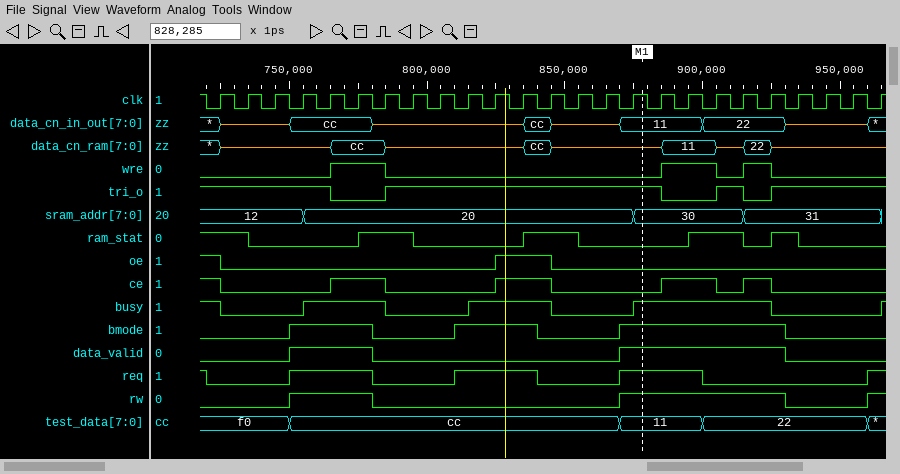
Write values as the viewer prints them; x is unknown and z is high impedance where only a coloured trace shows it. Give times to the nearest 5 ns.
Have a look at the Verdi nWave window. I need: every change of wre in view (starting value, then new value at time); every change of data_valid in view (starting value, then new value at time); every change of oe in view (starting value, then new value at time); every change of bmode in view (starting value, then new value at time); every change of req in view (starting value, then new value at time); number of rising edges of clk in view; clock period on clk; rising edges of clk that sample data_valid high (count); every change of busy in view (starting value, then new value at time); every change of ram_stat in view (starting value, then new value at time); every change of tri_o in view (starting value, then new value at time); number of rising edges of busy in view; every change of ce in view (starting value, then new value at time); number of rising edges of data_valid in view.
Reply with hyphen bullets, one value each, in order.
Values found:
- 0, 1 at 765 ns, 0 at 785 ns, 1 at 885 ns, 0 at 905 ns, 1 at 915 ns, 0 at 925 ns
- 0, 1 at 750 ns, 0 at 780 ns, 1 at 870 ns, 0 at 930 ns
- 1, 0 at 725 ns, 1 at 825 ns, 0 at 845 ns
- 0, 1 at 750 ns, 0 at 780 ns, 1 at 810 ns, 0 at 840 ns, 1 at 870 ns, 0 at 930 ns
- 1, 0 at 720 ns, 1 at 750 ns, 0 at 780 ns, 1 at 810 ns, 0 at 840 ns, 1 at 870 ns, 0 at 900 ns, 1 at 960 ns
- 25
- 10 ns
- 9
- 1, 0 at 725 ns, 1 at 755 ns, 0 at 785 ns, 1 at 815 ns, 0 at 845 ns, 1 at 875 ns, 0 at 925 ns, 1 at 965 ns
- 1, 0 at 735 ns, 1 at 775 ns, 0 at 795 ns, 1 at 835 ns, 0 at 855 ns, 1 at 895 ns, 0 at 915 ns, 1 at 925 ns, 0 at 935 ns
- 1, 0 at 765 ns, 1 at 785 ns, 0 at 885 ns, 1 at 905 ns, 0 at 915 ns, 1 at 925 ns
- 4
- 1, 0 at 725 ns, 1 at 765 ns, 0 at 785 ns, 1 at 825 ns, 0 at 845 ns, 1 at 885 ns, 0 at 905 ns, 1 at 915 ns, 0 at 925 ns
- 2
